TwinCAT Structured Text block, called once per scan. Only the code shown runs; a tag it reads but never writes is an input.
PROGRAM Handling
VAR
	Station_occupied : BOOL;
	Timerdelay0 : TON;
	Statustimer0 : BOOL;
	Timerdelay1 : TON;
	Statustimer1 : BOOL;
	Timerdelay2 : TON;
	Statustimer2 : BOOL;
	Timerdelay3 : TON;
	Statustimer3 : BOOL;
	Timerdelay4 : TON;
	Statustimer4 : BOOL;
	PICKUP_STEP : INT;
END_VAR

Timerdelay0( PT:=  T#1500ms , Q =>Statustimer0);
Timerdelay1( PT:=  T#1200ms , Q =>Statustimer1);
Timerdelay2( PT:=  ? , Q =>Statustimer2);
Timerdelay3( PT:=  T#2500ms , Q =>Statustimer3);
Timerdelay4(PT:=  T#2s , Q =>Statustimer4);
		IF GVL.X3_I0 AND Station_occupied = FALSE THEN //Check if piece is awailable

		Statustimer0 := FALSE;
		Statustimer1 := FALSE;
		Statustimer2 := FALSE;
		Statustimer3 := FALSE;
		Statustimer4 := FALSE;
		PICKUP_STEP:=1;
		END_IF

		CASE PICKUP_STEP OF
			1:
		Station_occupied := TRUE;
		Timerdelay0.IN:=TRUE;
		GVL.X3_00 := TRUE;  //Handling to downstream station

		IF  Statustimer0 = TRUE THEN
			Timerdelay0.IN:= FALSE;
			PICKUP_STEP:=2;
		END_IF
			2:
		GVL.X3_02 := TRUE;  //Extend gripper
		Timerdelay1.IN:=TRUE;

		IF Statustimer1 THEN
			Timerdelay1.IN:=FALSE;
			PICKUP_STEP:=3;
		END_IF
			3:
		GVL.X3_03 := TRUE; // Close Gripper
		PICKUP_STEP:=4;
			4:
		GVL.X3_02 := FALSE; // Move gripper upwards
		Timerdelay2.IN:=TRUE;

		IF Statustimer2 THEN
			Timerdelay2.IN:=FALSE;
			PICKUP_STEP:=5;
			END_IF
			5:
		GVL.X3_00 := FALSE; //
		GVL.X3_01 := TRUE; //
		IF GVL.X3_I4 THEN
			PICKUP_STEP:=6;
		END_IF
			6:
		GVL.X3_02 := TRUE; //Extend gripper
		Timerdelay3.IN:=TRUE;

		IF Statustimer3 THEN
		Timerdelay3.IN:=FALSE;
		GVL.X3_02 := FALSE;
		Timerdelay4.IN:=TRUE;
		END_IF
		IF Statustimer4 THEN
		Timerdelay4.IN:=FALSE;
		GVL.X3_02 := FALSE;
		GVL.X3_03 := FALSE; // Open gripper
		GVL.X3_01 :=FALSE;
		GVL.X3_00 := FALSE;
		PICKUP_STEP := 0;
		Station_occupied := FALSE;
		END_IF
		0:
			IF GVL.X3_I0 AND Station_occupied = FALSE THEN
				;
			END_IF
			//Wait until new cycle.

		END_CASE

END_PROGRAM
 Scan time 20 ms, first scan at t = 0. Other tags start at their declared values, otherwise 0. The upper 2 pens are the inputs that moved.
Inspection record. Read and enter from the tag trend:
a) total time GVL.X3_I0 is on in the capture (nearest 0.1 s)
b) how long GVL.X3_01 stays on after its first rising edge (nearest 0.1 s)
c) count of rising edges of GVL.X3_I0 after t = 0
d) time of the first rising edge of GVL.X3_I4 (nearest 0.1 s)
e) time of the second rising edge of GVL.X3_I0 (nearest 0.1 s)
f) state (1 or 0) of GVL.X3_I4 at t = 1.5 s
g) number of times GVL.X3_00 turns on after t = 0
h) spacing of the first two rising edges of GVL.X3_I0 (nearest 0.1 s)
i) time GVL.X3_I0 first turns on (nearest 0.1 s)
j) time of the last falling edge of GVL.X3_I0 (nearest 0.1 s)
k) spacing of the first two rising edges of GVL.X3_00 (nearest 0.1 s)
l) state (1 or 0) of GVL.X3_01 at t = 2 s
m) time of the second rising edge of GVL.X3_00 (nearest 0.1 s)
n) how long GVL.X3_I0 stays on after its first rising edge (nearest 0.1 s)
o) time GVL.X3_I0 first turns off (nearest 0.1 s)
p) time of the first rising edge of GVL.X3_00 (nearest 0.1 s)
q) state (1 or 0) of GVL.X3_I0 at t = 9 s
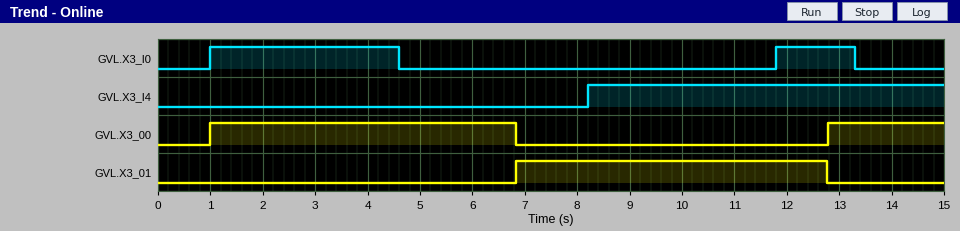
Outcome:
5.1 s
5.9 s
2
8.2 s
11.8 s
0
2
10.8 s
1.0 s
13.3 s
11.8 s
0
12.8 s
3.6 s
4.6 s
1.0 s
0
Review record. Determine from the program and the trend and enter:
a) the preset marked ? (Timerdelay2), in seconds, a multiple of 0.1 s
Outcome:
3.0 s
